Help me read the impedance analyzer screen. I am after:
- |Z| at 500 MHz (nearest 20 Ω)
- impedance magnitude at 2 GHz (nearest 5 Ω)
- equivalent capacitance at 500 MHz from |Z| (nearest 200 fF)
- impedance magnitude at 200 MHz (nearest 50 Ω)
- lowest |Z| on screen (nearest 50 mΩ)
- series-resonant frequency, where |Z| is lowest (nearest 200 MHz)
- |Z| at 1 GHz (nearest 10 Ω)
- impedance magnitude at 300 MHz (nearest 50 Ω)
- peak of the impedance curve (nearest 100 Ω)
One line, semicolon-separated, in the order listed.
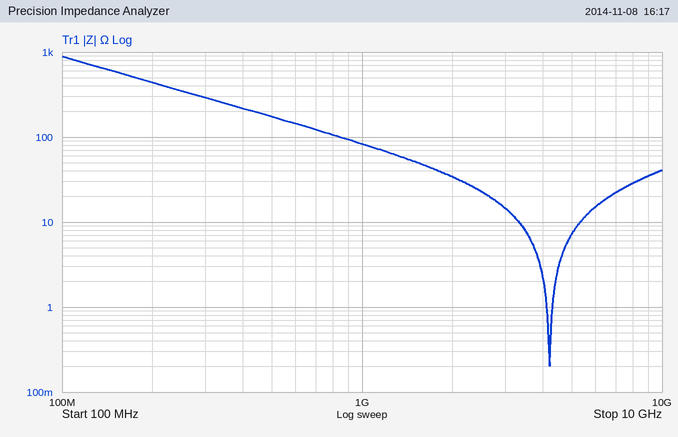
180 Ω; 35 Ω; 1.8 pF; 450 Ω; 200 mΩ; 4.2 GHz; 80 Ω; 300 Ω; 900 Ω
